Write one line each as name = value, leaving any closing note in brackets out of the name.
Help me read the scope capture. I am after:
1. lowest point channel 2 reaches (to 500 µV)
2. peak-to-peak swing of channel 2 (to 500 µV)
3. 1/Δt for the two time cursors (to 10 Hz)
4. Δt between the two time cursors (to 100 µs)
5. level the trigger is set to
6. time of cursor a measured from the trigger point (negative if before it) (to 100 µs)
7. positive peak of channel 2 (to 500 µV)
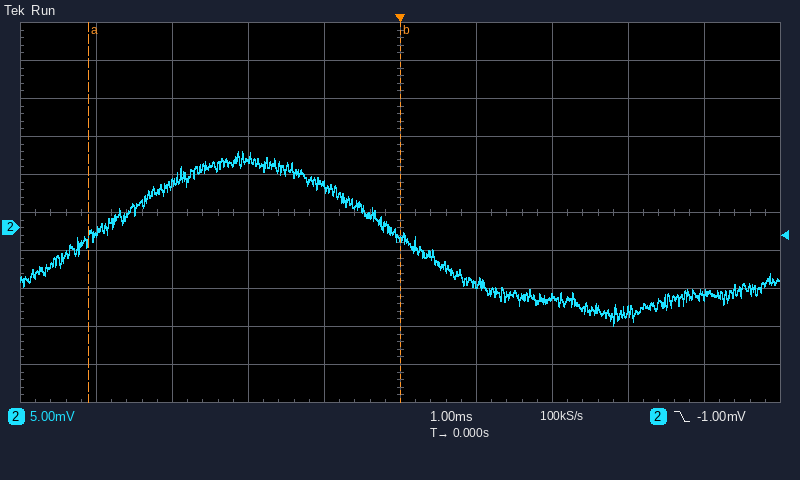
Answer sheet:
lowest point channel 2 reaches = -13.0 mV
peak-to-peak swing of channel 2 = 23.0 mV
1/Δt for the two time cursors = 240 Hz
Δt between the two time cursors = 4.1 ms
level the trigger is set to = -1.00 mV
time of cursor a measured from the trigger point (negative if before it) = -4.1 ms
positive peak of channel 2 = 10.0 mV
